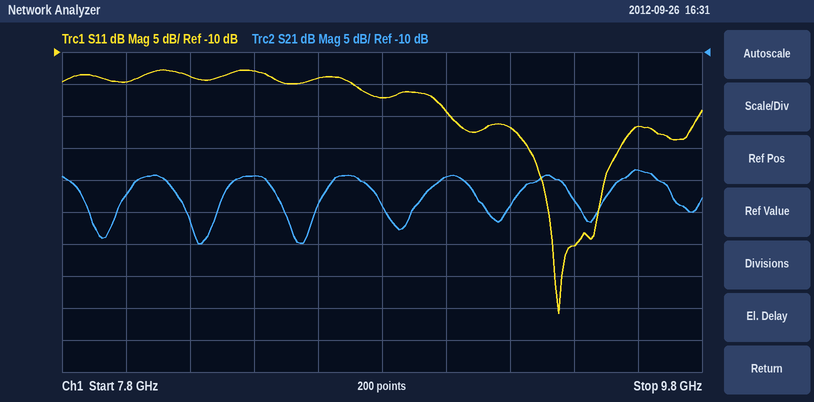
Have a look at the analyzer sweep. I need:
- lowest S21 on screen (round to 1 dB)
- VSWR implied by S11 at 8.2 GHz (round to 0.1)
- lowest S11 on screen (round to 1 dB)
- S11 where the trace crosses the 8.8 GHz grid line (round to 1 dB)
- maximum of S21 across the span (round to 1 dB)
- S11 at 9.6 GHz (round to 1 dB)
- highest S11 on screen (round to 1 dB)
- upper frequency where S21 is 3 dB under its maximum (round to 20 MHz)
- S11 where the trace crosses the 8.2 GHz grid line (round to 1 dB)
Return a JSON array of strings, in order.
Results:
["-40 dB", "1.5", "-51 dB", "-17 dB", "-28 dB", "-22 dB", "-13 dB", "9.70 GHz", "-14 dB"]
